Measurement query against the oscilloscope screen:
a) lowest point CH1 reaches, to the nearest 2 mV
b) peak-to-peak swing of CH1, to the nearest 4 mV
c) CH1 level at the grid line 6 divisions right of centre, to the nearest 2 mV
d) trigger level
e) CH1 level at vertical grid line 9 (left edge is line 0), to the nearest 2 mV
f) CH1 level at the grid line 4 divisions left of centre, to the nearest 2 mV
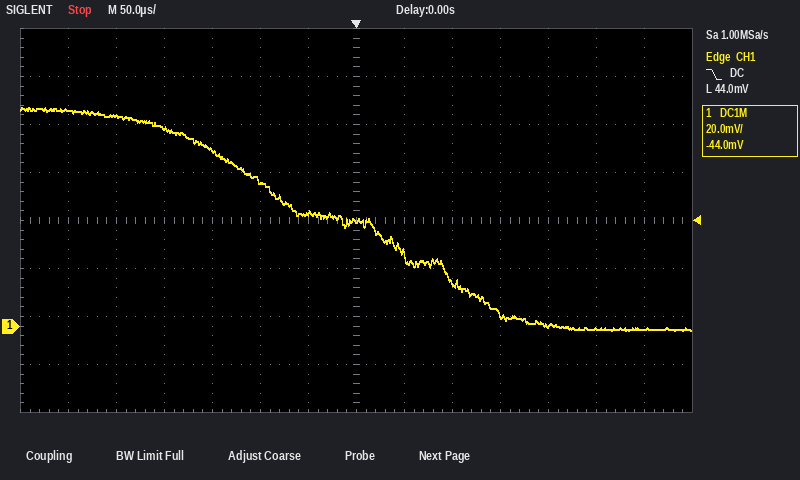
-2 mV
92 mV
-2 mV
44.0 mV
18 mV
82 mV
